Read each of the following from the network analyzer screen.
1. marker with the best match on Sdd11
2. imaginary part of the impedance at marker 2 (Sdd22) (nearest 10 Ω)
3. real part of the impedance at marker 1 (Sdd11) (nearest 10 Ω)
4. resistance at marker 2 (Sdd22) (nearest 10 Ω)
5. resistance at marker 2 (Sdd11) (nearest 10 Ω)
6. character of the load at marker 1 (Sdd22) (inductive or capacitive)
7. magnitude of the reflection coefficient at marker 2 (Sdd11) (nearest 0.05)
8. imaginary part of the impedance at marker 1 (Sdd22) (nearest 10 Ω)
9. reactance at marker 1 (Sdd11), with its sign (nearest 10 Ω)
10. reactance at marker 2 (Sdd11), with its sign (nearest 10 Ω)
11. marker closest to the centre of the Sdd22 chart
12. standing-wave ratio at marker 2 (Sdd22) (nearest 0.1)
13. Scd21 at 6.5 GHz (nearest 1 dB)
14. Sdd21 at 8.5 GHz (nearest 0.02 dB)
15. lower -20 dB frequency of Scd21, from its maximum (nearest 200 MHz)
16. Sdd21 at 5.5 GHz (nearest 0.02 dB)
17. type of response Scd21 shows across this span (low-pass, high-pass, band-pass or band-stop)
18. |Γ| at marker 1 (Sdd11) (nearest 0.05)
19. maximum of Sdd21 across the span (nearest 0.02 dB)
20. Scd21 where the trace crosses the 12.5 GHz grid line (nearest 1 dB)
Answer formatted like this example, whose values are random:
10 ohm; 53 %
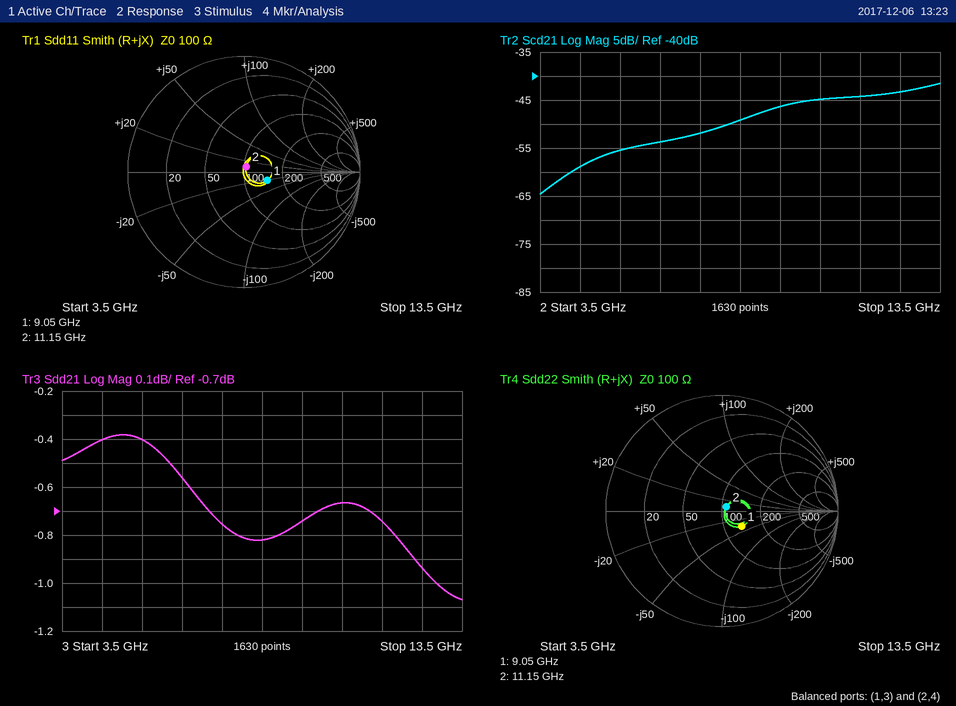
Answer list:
marker 2; +10 Ω; 150 Ω; 110 Ω; 100 Ω; capacitive; 0.05; -40 Ω; -20 Ω; +10 Ω; marker 2; 1.1; -54 dB; -0.82 dB; 4.0 GHz; -0.40 dB; high-pass; 0.20; -0.38 dB; -43 dB
